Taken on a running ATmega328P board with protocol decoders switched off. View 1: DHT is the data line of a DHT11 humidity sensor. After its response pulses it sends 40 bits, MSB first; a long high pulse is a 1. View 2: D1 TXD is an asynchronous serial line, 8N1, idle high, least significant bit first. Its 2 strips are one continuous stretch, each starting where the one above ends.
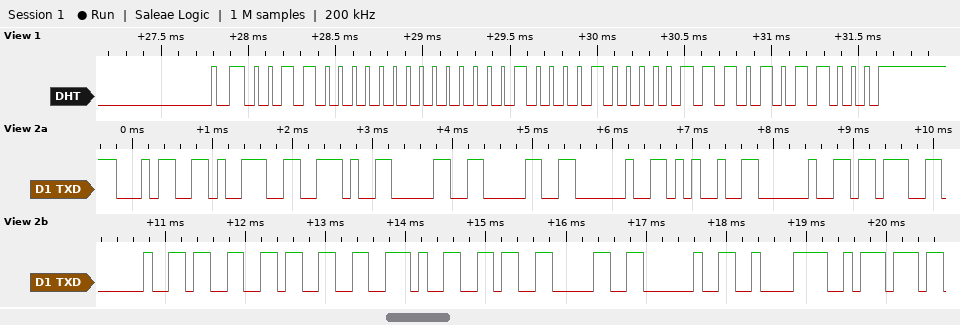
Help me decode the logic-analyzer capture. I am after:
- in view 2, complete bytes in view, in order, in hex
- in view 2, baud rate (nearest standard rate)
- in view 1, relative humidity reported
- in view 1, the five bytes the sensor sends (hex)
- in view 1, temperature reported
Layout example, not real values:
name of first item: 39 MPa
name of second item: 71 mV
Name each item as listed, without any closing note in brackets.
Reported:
in view 2, complete bytes in view, in order, in hex: 0x34 0x39 0x2E 0x30 0x30 0x20 0x25 0x20 0x3B 0x20 0x33 0x33 0x2E 0x36 0x30 0x20 0xC2 0xBA
in view 2, baud rate: 9600 baud
in view 1, relative humidity reported: 48 %
in view 1, the five bytes the sensor sends: 30 00 21 07 58
in view 1, temperature reported: 33.7 °C
